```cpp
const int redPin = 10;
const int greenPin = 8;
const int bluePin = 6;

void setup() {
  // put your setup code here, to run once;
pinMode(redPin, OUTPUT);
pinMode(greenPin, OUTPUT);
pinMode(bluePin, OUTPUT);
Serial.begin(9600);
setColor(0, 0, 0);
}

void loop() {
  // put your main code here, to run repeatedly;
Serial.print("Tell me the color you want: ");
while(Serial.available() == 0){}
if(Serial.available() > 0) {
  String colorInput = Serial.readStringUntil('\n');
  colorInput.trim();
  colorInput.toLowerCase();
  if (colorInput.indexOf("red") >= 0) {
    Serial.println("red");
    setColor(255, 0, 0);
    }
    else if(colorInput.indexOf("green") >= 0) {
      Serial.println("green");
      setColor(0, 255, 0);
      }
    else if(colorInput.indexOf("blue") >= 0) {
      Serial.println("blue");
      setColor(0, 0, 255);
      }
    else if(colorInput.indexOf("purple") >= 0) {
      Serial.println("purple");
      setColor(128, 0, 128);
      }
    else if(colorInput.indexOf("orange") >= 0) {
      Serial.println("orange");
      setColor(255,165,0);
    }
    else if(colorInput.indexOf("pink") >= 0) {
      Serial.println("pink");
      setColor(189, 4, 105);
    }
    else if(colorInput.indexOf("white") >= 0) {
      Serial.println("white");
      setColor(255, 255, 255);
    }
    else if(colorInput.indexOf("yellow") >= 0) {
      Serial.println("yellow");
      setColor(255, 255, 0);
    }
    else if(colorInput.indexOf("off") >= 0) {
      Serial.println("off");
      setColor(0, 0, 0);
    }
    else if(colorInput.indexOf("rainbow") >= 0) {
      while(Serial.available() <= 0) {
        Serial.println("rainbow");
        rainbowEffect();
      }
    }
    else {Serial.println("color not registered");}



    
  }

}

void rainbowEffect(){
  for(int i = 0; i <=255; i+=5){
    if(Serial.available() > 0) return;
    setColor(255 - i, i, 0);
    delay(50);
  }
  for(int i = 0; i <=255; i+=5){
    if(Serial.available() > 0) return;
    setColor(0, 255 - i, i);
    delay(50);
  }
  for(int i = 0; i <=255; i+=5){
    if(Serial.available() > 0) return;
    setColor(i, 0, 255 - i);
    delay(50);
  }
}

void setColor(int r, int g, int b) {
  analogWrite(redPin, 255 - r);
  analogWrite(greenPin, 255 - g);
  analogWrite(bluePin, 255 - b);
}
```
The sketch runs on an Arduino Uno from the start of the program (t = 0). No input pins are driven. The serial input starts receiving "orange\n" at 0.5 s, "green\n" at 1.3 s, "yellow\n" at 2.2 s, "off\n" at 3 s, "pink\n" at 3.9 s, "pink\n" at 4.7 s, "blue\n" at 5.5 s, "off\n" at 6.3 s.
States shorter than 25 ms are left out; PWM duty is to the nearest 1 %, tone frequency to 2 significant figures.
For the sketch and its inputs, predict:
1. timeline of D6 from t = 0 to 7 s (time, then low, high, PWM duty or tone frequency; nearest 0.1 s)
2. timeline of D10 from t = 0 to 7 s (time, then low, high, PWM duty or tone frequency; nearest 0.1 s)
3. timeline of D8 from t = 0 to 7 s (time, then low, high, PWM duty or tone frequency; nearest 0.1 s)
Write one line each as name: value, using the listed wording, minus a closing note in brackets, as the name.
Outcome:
timeline of D6 from t = 0 to 7 s: 0 s high; 3.9 s PWM 59 %; 5.5 s low; 6.3 s high
timeline of D10 from t = 0 to 7 s: 0 s high; 0.5 s low; 1.3 s high; 2.2 s low; 3 s high; 3.9 s PWM 26 %; 5.5 s high
timeline of D8 from t = 0 to 7 s: 0 s high; 0.5 s low; 3 s high
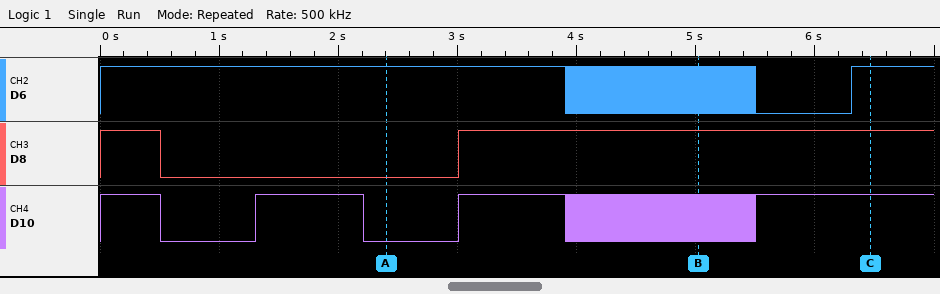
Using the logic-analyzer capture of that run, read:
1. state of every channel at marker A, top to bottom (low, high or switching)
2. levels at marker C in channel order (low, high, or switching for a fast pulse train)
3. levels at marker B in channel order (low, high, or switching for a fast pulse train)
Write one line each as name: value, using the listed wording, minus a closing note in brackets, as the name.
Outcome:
state of every channel at marker A, top to bottom: D6 high, D8 low, D10 low
levels at marker C in channel order: D6 high, D8 high, D10 high
levels at marker B in channel order: D6 switching, D8 high, D10 switching
